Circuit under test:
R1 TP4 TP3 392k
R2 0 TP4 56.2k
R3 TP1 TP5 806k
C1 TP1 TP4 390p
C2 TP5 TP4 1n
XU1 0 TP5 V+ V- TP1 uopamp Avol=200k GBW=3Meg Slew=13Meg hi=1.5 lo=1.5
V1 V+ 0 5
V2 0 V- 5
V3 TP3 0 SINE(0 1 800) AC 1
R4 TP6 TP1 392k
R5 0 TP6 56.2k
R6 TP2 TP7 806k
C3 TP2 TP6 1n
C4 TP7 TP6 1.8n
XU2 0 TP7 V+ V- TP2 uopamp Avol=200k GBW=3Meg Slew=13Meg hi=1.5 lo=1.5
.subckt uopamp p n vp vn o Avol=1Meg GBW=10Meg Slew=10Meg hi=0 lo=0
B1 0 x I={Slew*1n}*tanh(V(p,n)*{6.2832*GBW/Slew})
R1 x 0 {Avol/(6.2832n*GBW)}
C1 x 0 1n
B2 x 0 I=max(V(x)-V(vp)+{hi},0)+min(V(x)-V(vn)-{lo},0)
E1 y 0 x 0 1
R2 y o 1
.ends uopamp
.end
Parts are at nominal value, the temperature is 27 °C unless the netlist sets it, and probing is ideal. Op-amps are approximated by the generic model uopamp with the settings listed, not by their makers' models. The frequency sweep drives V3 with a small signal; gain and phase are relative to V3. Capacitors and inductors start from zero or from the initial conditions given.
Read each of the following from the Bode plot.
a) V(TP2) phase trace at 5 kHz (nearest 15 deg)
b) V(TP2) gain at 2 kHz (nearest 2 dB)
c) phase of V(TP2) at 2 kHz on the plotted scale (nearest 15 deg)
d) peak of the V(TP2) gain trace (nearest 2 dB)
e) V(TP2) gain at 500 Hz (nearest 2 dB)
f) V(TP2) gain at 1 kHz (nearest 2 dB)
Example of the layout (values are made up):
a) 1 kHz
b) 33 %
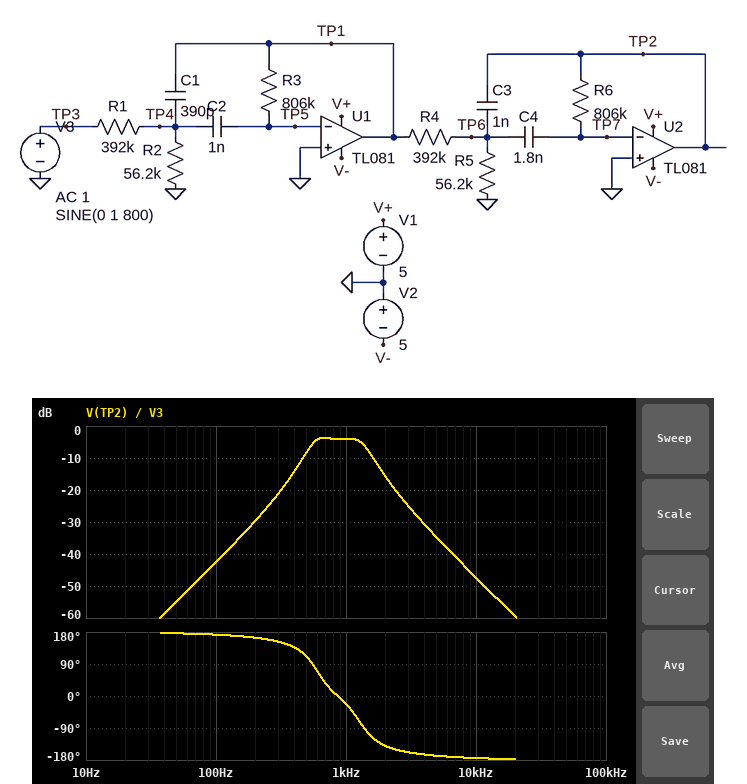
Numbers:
a) -165 deg
b) -16 dB
c) -135 deg
d) -4 dB
e) -8 dB
f) -4 dB
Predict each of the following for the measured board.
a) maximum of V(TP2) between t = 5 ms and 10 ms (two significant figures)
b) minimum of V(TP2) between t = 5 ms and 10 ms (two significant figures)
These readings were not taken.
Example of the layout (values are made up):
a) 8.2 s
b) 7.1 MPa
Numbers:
a) 630 mV
b) -630 mV
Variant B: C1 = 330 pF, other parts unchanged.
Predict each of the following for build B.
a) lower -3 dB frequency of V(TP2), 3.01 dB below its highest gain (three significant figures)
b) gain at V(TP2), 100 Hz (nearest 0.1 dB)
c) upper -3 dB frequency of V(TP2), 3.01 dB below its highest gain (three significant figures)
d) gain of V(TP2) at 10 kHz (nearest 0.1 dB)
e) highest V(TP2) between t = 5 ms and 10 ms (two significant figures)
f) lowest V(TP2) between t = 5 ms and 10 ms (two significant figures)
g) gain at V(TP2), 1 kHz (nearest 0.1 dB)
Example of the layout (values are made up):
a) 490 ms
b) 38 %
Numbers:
a) 523 Hz
b) -42.5 dB
c) 1.53 kHz
d) -45.9 dB
e) 590 mV
f) -590 mV
g) -4.9 dB
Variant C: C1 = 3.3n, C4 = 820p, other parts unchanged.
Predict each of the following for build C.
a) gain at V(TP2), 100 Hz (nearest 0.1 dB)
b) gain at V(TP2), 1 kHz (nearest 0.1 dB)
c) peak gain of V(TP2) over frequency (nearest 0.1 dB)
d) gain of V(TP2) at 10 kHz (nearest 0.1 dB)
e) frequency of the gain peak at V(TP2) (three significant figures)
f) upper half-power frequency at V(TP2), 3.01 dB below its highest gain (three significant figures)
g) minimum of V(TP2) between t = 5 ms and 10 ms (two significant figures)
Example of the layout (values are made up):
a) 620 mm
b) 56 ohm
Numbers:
a) -49.1 dB
b) -18.4 dB
c) -15.3 dB
d) -66.0 dB
e) 786 Hz
f) 995 Hz
g) -170 mV
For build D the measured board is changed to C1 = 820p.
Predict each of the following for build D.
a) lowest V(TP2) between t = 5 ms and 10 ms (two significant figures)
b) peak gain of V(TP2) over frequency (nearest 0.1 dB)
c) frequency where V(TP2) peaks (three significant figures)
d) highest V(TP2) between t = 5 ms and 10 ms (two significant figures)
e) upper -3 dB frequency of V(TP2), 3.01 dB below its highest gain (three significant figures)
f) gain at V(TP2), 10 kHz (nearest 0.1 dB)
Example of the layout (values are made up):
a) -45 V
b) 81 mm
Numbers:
a) -910 mV
b) -0.7 dB
c) 737 Hz
d) 910 mV
e) 958 Hz
f) -53.9 dB
